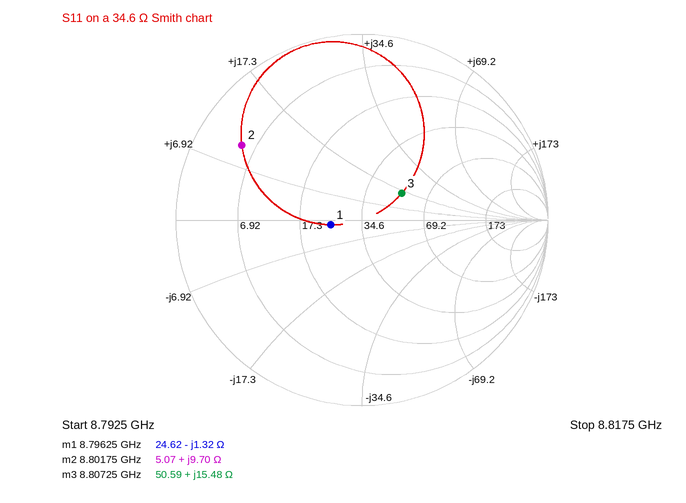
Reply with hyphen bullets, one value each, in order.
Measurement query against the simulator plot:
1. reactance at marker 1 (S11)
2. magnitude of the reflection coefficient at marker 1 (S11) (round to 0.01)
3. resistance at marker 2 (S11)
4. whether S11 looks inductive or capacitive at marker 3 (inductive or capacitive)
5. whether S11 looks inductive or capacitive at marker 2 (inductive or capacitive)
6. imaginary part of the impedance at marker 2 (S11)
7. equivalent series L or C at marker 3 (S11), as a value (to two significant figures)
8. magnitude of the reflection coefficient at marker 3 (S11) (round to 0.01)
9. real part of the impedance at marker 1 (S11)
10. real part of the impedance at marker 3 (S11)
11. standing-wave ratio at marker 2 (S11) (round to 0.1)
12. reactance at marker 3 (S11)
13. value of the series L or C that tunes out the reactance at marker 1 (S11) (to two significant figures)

- -1.32 Ω
- 0.17
- 5.07 Ω
- inductive
- inductive
- +9.70 Ω
- 280 pH
- 0.26
- 24.62 Ω
- 50.59 Ω
- 7.4
- +15.48 Ω
- 24 pH
